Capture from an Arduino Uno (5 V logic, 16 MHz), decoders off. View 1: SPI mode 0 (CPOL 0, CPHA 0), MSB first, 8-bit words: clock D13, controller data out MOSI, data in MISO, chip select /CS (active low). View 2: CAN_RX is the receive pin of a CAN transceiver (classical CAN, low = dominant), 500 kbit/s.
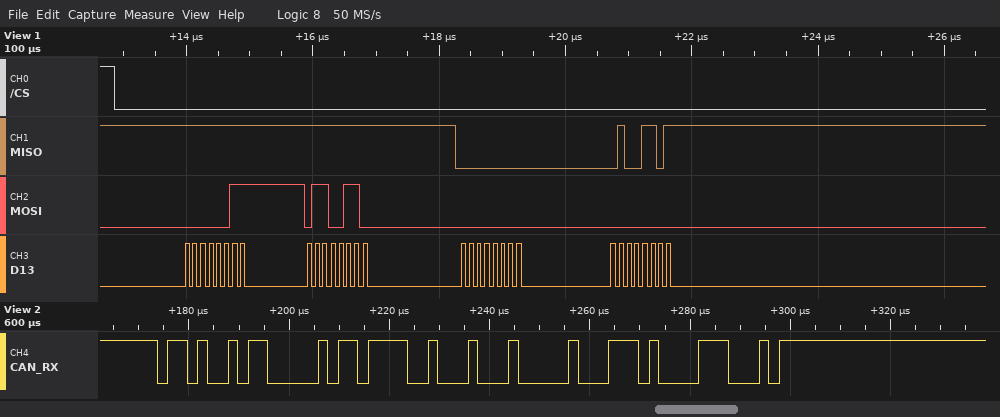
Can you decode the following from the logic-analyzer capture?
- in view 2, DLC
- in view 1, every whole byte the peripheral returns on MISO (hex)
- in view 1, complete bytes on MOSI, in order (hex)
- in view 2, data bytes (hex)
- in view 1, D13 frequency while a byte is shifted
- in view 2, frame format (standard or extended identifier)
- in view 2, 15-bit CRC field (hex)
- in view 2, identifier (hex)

3
0xFF 0xFF 0x00 0x4D
0x03 0x66 0x00 0x00
79 11 00
8 MHz
standard
0x7438
0x696
